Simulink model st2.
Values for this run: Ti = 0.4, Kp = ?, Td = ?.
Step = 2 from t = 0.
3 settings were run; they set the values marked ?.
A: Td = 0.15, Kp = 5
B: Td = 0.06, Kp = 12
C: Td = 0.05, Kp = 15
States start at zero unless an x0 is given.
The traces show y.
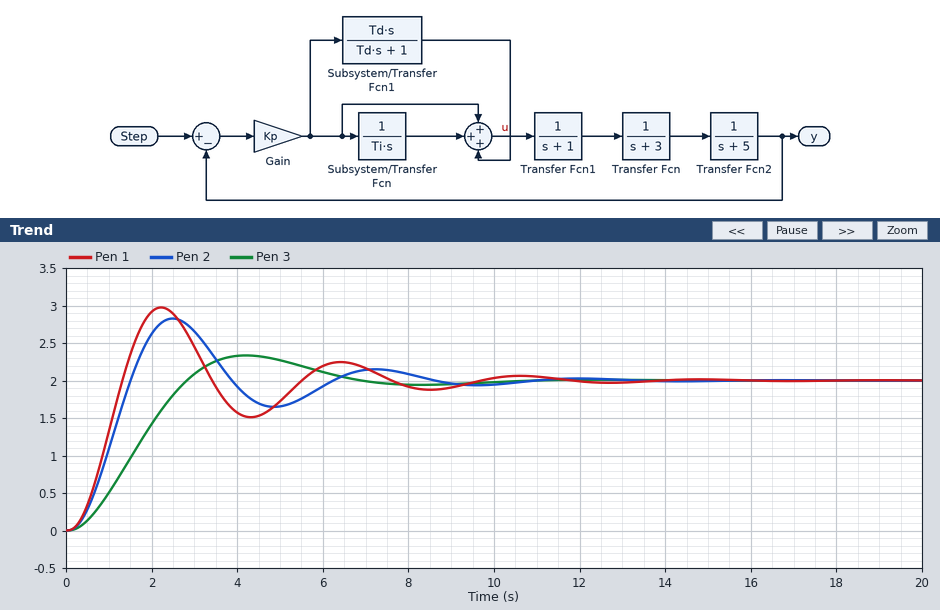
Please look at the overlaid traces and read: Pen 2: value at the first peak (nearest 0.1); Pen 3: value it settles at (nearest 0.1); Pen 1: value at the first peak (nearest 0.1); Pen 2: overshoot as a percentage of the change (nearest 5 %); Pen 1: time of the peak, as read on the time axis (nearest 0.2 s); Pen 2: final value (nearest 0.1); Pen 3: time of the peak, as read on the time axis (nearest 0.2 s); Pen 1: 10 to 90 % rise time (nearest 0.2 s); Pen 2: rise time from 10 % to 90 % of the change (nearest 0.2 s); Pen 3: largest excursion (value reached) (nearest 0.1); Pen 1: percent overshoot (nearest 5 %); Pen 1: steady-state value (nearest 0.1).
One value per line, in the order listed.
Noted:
2.8
2.0
3.0
40 %
2.2 s
2.0
4.2 s
0.8 s
1.0 s
2.3
50 %
2.0
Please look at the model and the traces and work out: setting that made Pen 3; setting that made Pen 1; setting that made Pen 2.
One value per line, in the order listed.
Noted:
A
C
B
